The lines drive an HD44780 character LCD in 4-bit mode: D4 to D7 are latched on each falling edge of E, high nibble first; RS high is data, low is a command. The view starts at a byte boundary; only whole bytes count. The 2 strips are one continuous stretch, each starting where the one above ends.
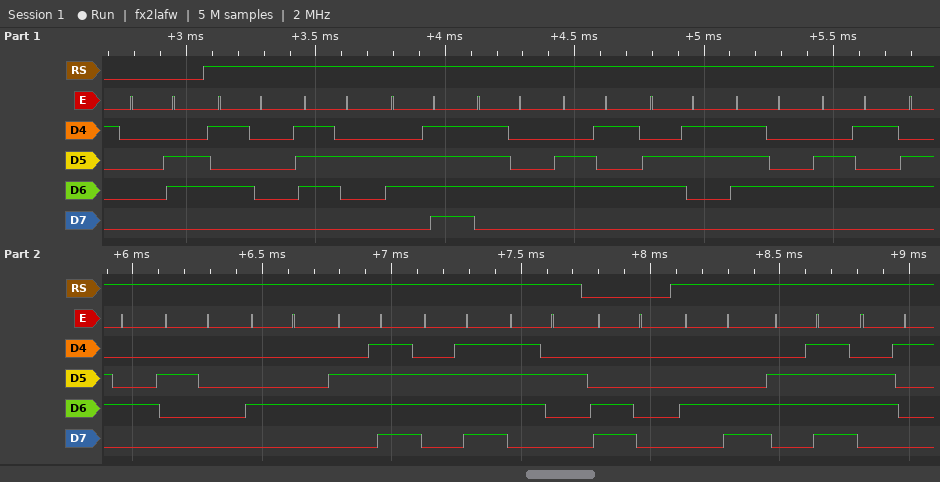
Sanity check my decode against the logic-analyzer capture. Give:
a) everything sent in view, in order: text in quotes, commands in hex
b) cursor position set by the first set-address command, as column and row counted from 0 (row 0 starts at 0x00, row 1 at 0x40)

0x06 "Protected Door" 0xC0 "Loa"
column 0, row 1
